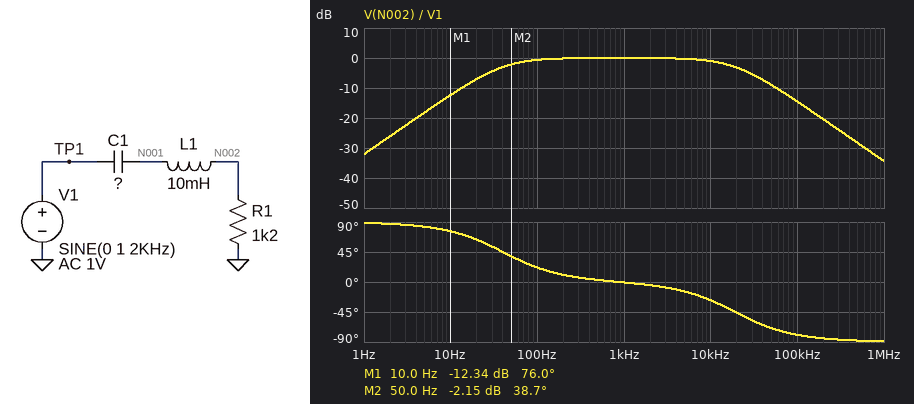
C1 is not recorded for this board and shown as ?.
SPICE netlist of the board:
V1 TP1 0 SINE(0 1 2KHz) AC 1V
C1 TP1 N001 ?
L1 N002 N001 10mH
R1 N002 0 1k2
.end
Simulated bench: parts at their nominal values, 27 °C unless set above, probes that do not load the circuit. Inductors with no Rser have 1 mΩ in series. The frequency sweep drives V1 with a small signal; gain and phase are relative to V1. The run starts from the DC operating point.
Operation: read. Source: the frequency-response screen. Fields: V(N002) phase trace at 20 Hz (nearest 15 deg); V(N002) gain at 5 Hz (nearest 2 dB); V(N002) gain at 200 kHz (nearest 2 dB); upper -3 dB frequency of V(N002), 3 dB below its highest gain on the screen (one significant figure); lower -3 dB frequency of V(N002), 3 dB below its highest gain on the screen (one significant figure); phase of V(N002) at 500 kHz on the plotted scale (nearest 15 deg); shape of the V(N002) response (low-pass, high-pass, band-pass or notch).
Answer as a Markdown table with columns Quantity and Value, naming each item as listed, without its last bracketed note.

| Quantity | Value |
|---|---|
| V(N002) phase trace at 20 Hz | 60 deg |
| V(N002) gain at 5 Hz | -18 dB |
| V(N002) gain at 200 kHz | -20 dB |
| upper -3 dB frequency of V(N002), 3 dB below its highest gain on the screen | 20 kHz |
| lower -3 dB frequency of V(N002), 3 dB below its highest gain on the screen | 40 Hz |
| phase of V(N002) at 500 kHz on the plotted scale | -90 deg |
| shape of the V(N002) response | band-pass |
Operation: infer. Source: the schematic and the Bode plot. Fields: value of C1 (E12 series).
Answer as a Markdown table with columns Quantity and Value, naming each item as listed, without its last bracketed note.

| Quantity | Value |
|---|---|
| value of C1 | 3.3 µF |
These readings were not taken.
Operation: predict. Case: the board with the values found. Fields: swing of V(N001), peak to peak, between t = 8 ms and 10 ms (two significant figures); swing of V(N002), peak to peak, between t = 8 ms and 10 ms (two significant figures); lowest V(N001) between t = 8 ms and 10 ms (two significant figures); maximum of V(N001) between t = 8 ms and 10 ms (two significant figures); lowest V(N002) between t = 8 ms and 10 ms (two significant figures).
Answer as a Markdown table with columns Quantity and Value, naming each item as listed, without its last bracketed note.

| Quantity | Value |
|---|---|
| swing of V(N001), peak to peak, between t = 8 ms and 10 ms | 2.0 V |
| swing of V(N002), peak to peak, between t = 8 ms and 10 ms | 2.0 V |
| lowest V(N001) between t = 8 ms and 10 ms | -1.0 V |
| maximum of V(N001) between t = 8 ms and 10 ms | 1.0 V |
| lowest V(N002) between t = 8 ms and 10 ms | -1.0 V |
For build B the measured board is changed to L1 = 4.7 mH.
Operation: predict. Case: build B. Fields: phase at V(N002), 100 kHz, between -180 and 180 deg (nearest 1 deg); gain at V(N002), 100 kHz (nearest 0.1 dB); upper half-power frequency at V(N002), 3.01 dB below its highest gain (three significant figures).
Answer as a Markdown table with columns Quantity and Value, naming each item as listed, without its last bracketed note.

| Quantity | Value |
|---|---|
| phase at V(N002), 100 kHz, between -180 and 180 deg | -68 deg |
| gain at V(N002), 100 kHz | -8.5 dB |
| upper half-power frequency at V(N002), 3.01 dB below its highest gain | 40.7 kHz |
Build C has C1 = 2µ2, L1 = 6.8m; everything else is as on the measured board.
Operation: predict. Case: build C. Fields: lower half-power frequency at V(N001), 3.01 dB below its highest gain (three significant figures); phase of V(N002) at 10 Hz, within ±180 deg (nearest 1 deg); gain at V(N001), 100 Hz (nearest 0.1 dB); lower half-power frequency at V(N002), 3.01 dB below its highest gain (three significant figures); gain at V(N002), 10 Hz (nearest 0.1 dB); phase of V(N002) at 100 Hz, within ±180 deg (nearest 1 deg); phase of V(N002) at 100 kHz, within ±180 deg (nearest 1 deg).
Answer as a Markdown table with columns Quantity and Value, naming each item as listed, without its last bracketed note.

| Quantity | Value |
|---|---|
| lower half-power frequency at V(N001), 3.01 dB below its highest gain | 60.4 Hz |
| phase of V(N002) at 10 Hz, within ±180 deg | 81 deg |
| gain at V(N001), 100 Hz | -1.3 dB |
| lower half-power frequency at V(N002), 3.01 dB below its highest gain | 60.2 Hz |
| gain at V(N002), 10 Hz | -15.7 dB |
| phase of V(N002) at 100 Hz, within ±180 deg | 31 deg |
| phase of V(N002) at 100 kHz, within ±180 deg | -74 deg |
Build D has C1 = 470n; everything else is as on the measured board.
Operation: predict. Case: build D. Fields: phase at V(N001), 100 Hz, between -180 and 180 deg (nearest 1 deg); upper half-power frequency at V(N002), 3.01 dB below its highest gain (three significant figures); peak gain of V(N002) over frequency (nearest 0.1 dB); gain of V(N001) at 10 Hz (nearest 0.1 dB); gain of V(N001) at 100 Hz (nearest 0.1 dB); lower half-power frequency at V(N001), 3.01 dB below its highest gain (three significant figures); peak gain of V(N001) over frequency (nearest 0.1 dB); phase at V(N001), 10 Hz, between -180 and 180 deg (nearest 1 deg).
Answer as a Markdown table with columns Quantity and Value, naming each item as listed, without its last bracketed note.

| Quantity | Value |
|---|---|
| phase at V(N001), 100 Hz, between -180 and 180 deg | 71 deg |
| upper half-power frequency at V(N002), 3.01 dB below its highest gain | 19.4 kHz |
| peak gain of V(N002) over frequency | 0 dB |
| gain of V(N001) at 10 Hz | -29.0 dB |
| gain of V(N001) at 100 Hz | -9.5 dB |
| lower half-power frequency at V(N001), 3.01 dB below its highest gain | 285 Hz |
| peak gain of V(N001) over frequency | 0.1 dB |
| phase at V(N001), 10 Hz, between -180 and 180 deg | 88 deg |
